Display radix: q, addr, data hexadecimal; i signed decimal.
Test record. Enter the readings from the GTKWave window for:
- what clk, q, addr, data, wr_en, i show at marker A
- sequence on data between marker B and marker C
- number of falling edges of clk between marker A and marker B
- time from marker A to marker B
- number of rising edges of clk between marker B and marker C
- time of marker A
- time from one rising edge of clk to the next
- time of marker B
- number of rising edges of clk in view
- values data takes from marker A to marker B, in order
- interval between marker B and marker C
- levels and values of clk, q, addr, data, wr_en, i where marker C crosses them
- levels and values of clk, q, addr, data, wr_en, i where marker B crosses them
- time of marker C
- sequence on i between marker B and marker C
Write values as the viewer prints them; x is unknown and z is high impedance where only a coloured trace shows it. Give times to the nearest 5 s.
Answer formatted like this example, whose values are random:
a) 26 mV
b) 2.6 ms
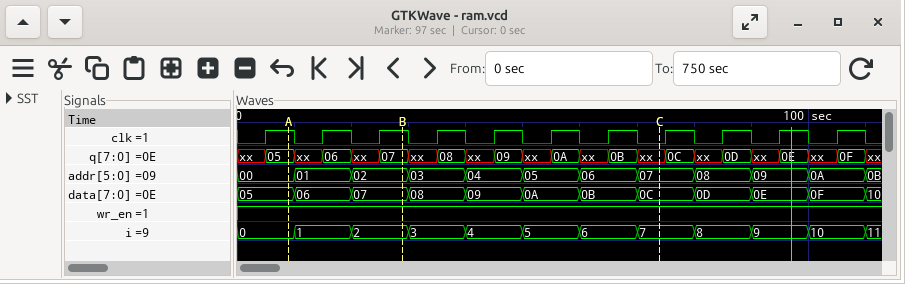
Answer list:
a) clk=1, q=05, addr=00, data=05, wr_en=1, i=0
b) 07, 08, 09, 0A, 0B, 0C
c) 2
d) 20 s
e) 4
f) 10 s
g) 10 s
h) 30 s
i) 11
j) 05, 06, 07
k) 45 s
l) clk=0, q=xx, addr=07, data=0C, wr_en=1, i=7
m) clk=1, q=07, addr=02, data=07, wr_en=1, i=2
n) 75 s
o) 2, 3, 4, 5, 6, 7
